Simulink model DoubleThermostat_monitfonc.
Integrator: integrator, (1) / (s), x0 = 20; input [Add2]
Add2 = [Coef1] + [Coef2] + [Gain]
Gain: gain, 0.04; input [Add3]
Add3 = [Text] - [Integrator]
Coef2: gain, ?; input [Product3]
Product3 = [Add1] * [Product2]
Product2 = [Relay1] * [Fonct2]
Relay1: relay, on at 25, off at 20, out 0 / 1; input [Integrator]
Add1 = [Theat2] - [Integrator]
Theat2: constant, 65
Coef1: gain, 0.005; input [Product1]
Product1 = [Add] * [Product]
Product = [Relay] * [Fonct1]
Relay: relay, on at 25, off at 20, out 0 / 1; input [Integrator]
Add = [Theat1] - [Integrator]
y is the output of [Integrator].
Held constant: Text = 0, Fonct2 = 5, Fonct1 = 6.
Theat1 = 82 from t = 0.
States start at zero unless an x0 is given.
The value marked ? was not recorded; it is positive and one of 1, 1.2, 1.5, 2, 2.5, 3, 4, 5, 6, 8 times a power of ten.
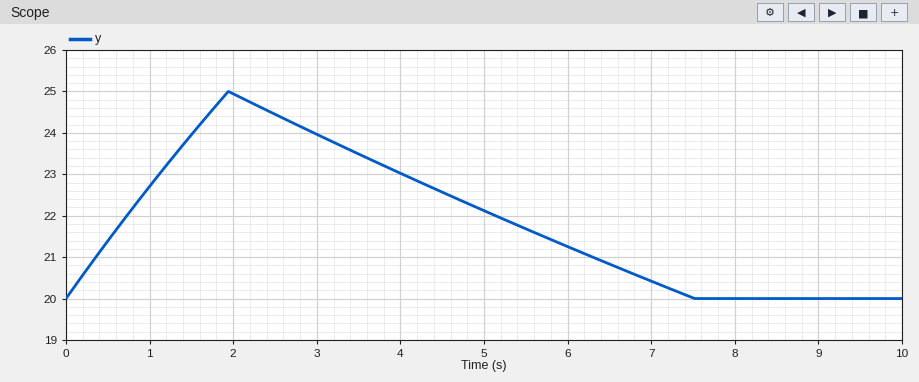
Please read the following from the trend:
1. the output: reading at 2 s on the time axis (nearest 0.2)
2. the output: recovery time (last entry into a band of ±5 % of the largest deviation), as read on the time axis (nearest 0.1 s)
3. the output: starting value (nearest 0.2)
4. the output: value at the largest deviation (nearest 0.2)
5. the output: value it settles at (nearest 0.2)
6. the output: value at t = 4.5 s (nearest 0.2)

25.0
7.2 s
20.0
25.0
20.0
22.6
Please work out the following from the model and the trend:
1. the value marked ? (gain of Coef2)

0.008
